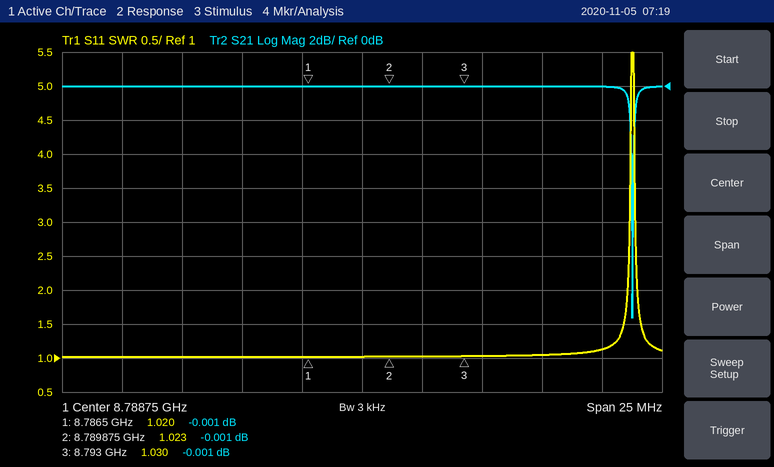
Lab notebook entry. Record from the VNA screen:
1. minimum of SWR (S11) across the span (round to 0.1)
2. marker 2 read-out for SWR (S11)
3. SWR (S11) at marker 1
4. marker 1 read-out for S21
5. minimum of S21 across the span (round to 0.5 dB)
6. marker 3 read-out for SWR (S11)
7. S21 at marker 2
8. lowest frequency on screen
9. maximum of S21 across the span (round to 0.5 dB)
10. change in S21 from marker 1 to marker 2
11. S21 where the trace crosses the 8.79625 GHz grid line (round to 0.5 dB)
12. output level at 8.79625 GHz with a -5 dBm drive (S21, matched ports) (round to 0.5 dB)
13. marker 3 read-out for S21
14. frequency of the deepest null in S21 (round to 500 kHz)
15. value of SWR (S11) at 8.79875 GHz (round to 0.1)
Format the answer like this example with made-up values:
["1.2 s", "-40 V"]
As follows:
["1.0", "1.023", "1.020", "-0.001 dB", "-13.5 dB", "1.030", "-0.001 dB", "8.77625 GHz", "0.0 dB", "0.000 dB", "0.0 dB", "-5.0 dBm", "-0.001 dB", "8.8000 GHz", "1.1"]
